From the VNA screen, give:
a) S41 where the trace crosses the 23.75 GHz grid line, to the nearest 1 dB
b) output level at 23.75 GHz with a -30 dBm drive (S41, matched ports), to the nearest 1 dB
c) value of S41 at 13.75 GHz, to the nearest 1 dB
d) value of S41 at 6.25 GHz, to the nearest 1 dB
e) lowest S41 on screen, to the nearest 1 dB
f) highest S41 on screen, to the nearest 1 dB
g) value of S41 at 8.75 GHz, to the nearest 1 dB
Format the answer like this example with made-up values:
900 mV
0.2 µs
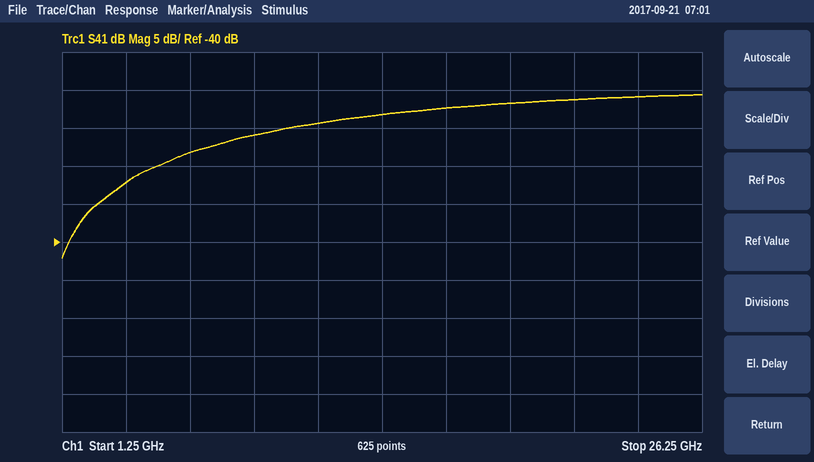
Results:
-21 dB
-51 dBm
-23 dB
-28 dB
-42 dB
-21 dB
-26 dB
